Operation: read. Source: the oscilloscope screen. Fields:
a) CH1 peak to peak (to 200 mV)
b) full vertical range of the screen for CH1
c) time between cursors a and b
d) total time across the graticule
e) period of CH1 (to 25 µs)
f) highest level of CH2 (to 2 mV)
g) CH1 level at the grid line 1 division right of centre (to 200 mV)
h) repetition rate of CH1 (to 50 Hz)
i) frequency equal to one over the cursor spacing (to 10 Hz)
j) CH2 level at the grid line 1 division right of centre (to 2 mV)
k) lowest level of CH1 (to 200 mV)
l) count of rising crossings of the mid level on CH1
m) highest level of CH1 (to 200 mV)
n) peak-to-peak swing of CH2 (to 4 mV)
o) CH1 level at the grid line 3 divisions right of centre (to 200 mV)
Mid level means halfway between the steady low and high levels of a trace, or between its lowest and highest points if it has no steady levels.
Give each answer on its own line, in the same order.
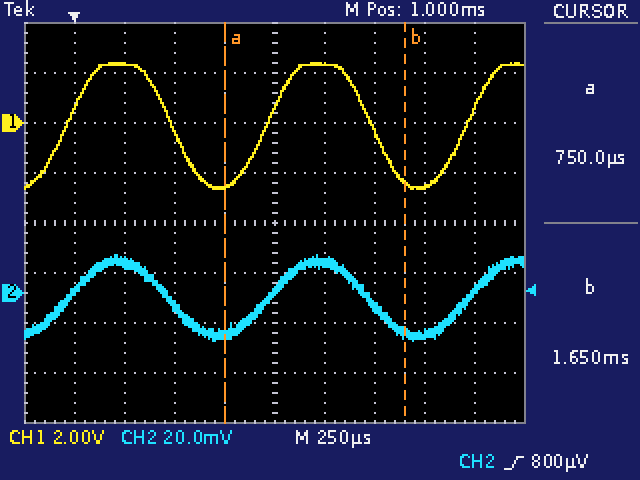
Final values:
5.0 V
16 V
900 µs
2.5 ms
1.000 ms
16 mV
2.4 V
1.00 kHz
1.11 kHz
12 mV
-2.6 V
3
2.4 V
36 mV
-2.6 V
